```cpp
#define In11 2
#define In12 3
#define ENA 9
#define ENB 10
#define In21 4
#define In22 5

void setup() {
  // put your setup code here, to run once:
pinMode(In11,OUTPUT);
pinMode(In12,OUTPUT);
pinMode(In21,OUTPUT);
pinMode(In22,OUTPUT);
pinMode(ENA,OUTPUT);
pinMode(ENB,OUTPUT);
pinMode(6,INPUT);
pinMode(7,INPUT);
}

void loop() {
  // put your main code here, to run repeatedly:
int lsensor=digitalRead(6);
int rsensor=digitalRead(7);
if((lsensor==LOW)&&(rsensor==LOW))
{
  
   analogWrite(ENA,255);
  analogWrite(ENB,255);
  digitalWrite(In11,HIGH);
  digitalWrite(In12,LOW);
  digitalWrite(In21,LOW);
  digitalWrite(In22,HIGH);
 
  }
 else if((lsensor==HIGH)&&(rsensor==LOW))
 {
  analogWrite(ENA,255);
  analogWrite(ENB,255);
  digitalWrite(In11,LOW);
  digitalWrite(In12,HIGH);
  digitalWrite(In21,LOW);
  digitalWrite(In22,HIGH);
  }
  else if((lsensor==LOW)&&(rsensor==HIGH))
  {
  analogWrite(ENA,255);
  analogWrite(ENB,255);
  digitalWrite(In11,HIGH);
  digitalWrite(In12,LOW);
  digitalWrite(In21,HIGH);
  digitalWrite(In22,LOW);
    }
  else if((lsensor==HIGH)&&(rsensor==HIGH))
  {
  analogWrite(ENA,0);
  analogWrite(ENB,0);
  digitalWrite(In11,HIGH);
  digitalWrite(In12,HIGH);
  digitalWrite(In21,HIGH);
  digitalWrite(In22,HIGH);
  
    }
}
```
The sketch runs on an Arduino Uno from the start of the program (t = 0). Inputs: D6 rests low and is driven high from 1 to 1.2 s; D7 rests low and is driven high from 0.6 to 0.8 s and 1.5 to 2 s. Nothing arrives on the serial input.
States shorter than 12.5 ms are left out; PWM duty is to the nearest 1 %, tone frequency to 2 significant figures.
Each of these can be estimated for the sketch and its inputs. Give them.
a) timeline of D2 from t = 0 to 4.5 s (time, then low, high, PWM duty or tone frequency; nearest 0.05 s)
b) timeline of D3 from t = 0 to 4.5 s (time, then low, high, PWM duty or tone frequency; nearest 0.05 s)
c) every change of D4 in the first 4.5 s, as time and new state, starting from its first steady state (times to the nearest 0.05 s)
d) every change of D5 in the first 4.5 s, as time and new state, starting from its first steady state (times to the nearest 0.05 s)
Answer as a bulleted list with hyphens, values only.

- 0 s high; 1 s low; 1.2 s high
- 0 s low; 1 s high; 1.2 s low
- 0 s low; 0.6 s high; 0.8 s low; 1.5 s high; 2 s low
- 0 s high; 0.6 s low; 0.8 s high; 1.5 s low; 2 s high
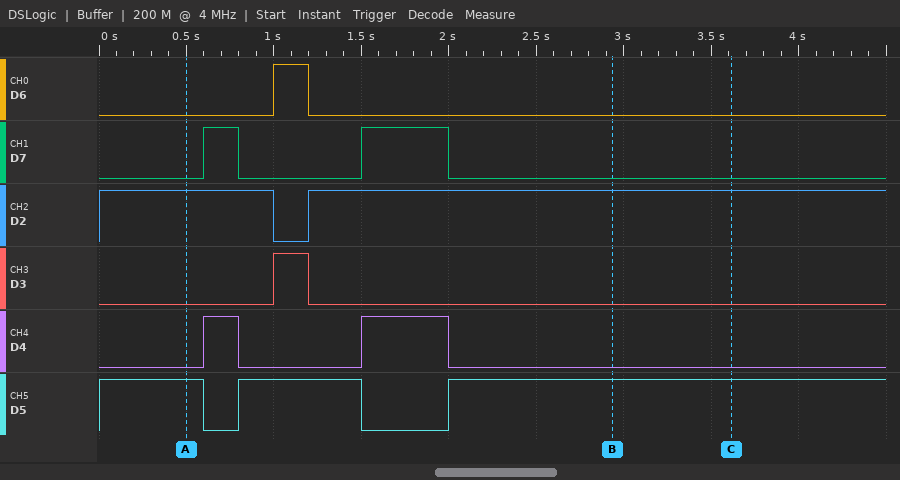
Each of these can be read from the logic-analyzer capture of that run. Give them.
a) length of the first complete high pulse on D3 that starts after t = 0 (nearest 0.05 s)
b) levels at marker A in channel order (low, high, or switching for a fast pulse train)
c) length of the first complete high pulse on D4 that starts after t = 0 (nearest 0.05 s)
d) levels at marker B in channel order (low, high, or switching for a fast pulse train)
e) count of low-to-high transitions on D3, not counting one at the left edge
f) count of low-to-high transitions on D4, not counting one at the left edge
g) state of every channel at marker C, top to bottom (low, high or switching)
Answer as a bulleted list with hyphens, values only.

- 0.20 s
- D6 low, D7 low, D2 high, D3 low, D4 low, D5 high
- 0.20 s
- D6 low, D7 low, D2 high, D3 low, D4 low, D5 high
- 1
- 2
- D6 low, D7 low, D2 high, D3 low, D4 low, D5 high
